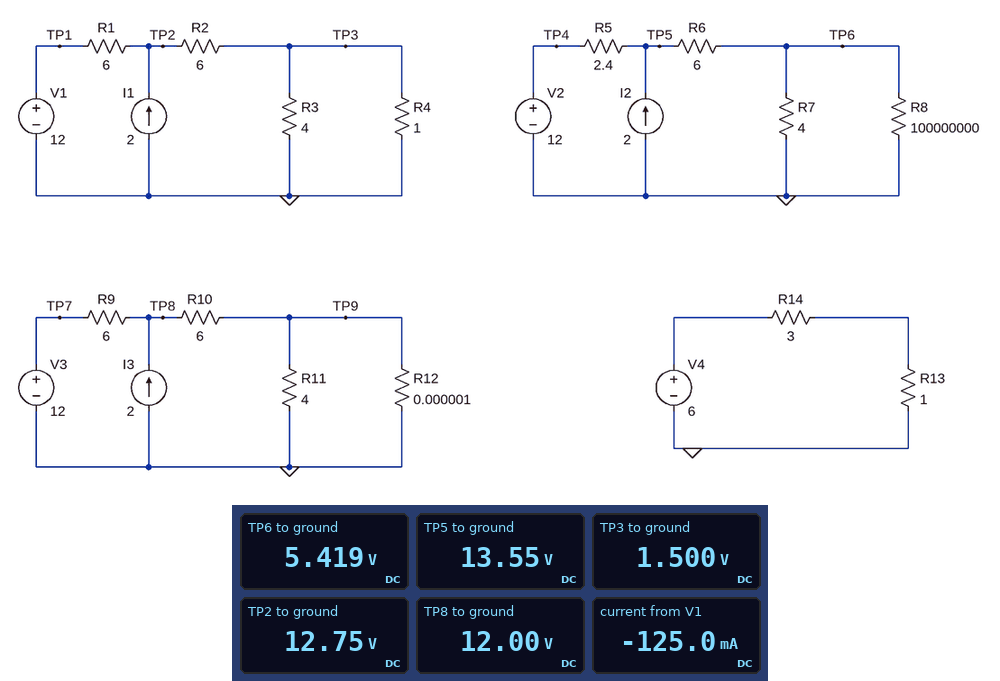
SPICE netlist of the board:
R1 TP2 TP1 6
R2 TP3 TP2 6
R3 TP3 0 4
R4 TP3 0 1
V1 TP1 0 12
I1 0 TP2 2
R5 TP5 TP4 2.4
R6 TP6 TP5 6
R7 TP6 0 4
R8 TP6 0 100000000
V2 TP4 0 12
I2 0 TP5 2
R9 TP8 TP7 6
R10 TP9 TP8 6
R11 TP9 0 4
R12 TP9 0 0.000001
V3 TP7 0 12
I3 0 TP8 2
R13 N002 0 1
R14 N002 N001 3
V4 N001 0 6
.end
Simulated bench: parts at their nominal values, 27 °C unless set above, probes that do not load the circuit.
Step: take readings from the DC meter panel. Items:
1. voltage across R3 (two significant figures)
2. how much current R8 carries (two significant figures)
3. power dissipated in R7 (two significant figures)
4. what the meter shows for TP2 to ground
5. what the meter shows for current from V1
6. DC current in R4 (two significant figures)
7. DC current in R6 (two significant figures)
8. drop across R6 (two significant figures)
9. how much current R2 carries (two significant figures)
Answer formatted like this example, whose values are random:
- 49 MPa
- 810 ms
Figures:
- 1.5 V
- 54 nA
- 7.3 W
- 12.75 V
- -125.0 mA
- 1.5 A
- 1.4 A
- 8.1 V
- 1.9 A
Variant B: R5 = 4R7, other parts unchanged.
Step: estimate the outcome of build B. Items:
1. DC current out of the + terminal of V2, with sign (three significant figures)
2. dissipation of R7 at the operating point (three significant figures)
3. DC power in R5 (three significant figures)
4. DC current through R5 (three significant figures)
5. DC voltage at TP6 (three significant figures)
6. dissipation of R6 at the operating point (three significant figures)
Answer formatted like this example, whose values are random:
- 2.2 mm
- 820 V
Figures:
- -544 mA
- 8.48 W
- 1.39 W
- 544 mA
- 5.82 V
- 12.7 W
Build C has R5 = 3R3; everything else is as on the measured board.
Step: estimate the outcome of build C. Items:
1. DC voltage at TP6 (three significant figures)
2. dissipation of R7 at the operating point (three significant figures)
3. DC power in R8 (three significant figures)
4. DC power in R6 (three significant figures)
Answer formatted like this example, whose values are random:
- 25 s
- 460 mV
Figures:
- 5.59 V
- 7.82 W
- 313 nW
- 11.7 W
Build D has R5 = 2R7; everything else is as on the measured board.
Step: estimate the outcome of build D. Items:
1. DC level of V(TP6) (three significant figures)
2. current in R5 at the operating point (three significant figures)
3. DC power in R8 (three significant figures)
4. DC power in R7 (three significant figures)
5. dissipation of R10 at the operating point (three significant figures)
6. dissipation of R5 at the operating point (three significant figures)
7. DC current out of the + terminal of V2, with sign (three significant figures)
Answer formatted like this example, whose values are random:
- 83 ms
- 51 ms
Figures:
- 5.48 V
- 630 mA
- 300 nW
- 7.51 W
- 24.0 W
- 1.07 W
- -630 mA
